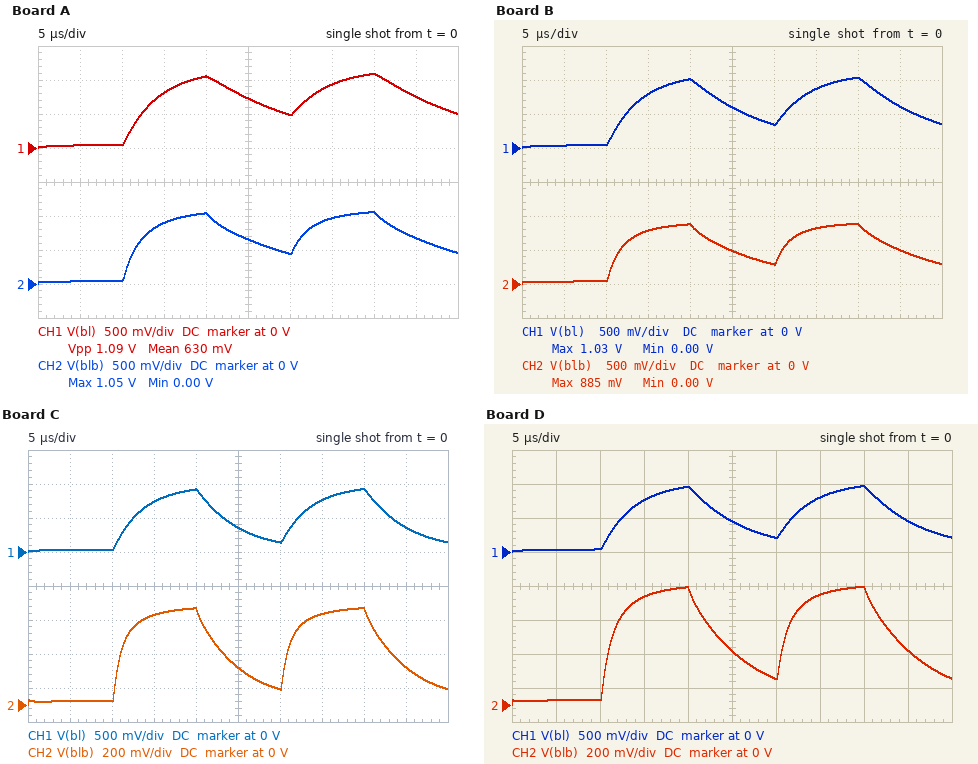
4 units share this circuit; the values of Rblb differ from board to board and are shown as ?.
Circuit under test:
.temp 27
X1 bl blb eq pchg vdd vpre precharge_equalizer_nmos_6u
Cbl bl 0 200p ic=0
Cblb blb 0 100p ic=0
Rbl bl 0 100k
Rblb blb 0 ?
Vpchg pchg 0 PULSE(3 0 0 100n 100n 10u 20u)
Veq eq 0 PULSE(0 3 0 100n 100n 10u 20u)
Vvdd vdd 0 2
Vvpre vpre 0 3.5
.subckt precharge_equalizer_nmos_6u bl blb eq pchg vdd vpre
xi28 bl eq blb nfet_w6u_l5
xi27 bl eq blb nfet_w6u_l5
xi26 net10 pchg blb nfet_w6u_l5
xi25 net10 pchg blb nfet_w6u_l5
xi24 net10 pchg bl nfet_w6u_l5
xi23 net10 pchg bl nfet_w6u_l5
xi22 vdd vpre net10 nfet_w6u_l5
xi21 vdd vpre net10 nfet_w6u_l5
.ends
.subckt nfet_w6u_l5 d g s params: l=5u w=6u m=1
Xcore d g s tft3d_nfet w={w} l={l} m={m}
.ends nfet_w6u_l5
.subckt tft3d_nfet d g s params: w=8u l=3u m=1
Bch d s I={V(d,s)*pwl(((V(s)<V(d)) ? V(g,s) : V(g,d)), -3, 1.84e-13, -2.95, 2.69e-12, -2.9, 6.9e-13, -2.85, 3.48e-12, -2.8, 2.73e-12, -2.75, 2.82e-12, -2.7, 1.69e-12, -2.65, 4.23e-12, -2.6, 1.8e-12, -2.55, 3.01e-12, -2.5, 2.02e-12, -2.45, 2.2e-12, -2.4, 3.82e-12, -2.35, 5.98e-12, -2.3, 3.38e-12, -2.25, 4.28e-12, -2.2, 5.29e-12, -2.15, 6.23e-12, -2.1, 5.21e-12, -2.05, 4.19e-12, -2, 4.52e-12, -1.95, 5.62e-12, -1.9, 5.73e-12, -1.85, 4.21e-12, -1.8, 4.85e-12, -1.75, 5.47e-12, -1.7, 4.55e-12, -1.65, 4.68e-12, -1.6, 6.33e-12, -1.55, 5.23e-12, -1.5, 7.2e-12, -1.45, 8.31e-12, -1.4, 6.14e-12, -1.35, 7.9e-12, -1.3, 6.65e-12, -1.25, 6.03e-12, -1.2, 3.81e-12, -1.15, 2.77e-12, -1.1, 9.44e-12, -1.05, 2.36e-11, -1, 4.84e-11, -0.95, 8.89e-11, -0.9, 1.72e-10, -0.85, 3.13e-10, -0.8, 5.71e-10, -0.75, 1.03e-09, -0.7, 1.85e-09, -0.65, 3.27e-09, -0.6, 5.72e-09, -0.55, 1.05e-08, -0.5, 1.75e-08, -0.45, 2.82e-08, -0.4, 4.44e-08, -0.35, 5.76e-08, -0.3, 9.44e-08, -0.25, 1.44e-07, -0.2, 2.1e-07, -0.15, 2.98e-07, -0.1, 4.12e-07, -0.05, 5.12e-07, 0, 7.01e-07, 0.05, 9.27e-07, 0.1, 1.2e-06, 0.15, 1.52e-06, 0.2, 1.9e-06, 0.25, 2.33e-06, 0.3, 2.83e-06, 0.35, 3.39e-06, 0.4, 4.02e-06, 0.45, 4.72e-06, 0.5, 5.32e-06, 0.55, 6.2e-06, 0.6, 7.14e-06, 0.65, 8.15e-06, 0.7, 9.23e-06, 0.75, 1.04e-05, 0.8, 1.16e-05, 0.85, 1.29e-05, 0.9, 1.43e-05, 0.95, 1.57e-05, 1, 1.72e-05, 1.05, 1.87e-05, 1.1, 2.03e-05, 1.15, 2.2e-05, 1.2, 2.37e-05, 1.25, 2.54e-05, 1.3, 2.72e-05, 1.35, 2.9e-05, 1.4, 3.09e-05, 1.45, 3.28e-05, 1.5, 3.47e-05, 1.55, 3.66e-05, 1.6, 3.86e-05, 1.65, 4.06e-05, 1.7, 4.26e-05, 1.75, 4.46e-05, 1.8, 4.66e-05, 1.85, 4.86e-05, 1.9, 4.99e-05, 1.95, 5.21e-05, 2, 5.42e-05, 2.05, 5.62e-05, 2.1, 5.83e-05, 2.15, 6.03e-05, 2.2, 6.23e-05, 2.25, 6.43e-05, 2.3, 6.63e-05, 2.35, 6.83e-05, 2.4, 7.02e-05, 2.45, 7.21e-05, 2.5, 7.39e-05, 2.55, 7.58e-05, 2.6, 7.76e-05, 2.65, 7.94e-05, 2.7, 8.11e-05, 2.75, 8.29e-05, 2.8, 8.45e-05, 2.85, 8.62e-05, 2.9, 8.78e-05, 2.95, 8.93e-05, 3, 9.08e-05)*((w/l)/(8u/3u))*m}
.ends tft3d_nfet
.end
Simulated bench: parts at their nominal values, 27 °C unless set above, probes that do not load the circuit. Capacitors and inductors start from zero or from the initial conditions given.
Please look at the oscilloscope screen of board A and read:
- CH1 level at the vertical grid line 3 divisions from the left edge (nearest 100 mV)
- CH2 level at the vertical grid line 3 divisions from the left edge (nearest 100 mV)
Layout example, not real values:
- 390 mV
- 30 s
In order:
- 800 mV
- 900 mV
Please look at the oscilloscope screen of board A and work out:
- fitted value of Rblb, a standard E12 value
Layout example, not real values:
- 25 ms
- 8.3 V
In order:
- 68 kΩ
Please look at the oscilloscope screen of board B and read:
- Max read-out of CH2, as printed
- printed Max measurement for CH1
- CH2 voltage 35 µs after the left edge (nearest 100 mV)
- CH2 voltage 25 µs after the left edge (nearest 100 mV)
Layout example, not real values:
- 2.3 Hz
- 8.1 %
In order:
- 885 mV
- 1.03 V
- 800 mV
- 500 mV
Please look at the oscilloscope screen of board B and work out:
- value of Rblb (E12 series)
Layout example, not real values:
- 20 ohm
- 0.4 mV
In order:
- 39 kΩ
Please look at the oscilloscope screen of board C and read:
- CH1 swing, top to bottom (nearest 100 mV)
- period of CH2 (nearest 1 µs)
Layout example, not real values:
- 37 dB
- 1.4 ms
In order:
- 900 mV
- 20 µs
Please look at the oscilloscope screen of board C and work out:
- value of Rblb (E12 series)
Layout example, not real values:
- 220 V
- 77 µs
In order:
- 15 kΩ
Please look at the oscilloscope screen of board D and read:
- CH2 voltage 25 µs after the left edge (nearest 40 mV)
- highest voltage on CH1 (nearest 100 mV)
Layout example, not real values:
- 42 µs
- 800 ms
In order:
- 320 mV
- 1.0 V
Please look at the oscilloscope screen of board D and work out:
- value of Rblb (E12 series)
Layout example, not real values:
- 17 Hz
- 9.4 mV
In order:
- 22 kΩ
